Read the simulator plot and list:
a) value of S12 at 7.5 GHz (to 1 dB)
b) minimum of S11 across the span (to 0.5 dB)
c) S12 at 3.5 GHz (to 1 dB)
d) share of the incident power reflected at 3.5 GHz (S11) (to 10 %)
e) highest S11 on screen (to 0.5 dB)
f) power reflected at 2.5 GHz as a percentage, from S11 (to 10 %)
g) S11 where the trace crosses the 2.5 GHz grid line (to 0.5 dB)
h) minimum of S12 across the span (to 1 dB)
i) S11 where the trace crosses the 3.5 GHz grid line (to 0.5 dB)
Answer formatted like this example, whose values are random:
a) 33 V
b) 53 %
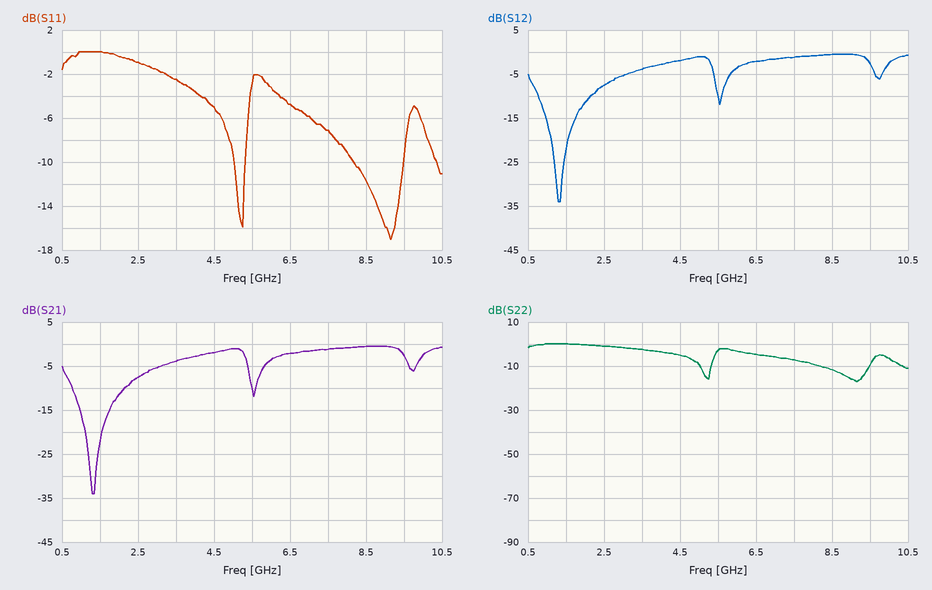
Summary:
a) -1 dB
b) -17.0 dB
c) -4 dB
d) 60 %
e) 0.0 dB
f) 80 %
g) -1.0 dB
h) -34 dB
i) -2.5 dB
